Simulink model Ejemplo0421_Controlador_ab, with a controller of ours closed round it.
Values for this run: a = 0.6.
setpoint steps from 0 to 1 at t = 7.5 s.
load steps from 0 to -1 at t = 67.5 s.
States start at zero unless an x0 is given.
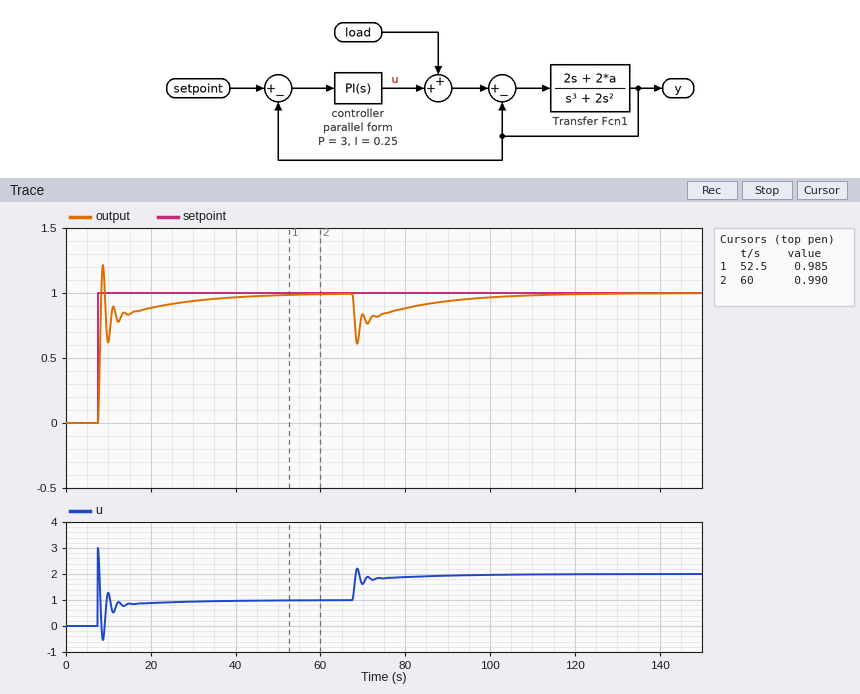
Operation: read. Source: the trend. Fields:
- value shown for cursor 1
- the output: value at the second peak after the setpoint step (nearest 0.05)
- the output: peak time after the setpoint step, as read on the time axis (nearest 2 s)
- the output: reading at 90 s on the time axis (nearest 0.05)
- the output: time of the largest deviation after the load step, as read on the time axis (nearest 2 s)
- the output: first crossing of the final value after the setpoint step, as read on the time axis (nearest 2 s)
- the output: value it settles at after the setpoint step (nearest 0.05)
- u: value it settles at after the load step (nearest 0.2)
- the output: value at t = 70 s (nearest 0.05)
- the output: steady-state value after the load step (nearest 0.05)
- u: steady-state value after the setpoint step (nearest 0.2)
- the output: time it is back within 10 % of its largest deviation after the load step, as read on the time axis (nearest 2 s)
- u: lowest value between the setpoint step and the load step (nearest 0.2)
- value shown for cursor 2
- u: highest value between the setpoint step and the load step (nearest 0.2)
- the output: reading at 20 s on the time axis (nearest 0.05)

0.985
0.90
8 s
0.95
68 s
8 s
1.00
2.0
0.85
1.00
1.0
98 s
-0.6
0.990
3.0
0.90
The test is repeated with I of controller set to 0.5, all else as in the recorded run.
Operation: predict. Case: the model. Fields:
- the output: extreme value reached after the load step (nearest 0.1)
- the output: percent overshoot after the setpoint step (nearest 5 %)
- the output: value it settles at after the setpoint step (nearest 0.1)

0.6
25 %
1.0
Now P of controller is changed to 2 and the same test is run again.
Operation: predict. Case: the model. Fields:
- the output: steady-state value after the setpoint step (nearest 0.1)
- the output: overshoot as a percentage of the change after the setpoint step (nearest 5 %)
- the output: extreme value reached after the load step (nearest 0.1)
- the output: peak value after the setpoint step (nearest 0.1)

1.0
10 %
0.5
1.1
